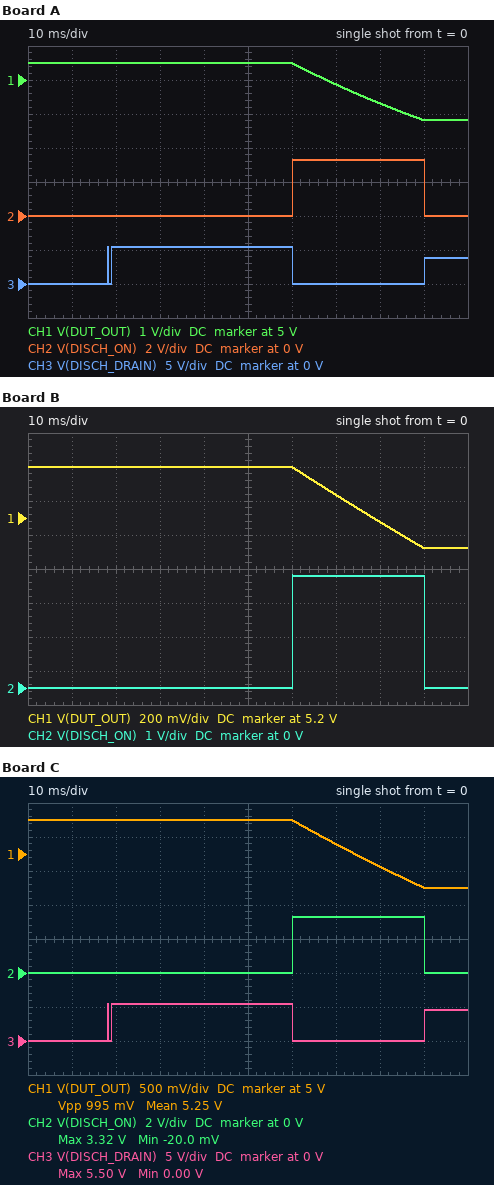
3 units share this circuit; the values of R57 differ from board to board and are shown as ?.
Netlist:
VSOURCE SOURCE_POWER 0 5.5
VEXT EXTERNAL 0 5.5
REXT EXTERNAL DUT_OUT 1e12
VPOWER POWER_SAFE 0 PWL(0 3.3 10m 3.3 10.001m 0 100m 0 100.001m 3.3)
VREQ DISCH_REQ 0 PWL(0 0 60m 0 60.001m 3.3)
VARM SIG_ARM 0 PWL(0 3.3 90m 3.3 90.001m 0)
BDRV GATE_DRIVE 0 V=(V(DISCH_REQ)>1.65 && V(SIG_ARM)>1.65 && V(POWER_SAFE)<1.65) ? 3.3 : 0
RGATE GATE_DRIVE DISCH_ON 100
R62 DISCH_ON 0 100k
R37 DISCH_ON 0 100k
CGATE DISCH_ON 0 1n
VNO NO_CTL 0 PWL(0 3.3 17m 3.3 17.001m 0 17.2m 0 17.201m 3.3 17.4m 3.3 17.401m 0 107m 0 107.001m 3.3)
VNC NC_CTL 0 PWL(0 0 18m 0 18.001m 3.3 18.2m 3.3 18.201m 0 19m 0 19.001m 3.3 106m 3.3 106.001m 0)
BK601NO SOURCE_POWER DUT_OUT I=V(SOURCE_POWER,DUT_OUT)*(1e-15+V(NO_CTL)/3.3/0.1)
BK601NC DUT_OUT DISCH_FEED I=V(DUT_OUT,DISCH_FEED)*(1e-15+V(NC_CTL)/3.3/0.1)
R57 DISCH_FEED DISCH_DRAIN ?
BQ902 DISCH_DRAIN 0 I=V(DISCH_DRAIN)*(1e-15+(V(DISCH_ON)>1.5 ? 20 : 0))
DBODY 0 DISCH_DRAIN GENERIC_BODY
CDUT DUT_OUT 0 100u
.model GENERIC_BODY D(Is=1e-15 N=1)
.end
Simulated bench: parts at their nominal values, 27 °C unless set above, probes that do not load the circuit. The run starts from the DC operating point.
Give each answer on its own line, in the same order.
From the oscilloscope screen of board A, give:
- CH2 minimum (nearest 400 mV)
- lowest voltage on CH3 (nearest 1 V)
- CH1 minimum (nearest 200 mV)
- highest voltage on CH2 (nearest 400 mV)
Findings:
0 V
0 V
3.8 V
3.2 V
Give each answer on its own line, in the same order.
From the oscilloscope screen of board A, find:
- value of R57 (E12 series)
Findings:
820 Ω
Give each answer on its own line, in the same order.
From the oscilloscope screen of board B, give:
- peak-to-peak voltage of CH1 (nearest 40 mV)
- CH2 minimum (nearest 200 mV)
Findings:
480 mV
0 V
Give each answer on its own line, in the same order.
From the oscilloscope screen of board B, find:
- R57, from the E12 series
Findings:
3.3 kΩ
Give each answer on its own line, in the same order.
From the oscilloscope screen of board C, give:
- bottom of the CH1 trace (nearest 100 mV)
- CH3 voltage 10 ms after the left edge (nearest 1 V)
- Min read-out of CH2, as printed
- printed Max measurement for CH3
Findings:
4.5 V
0 V
-20.0 mV
5.50 V
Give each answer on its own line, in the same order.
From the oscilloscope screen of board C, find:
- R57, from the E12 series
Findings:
1.5 kΩ
